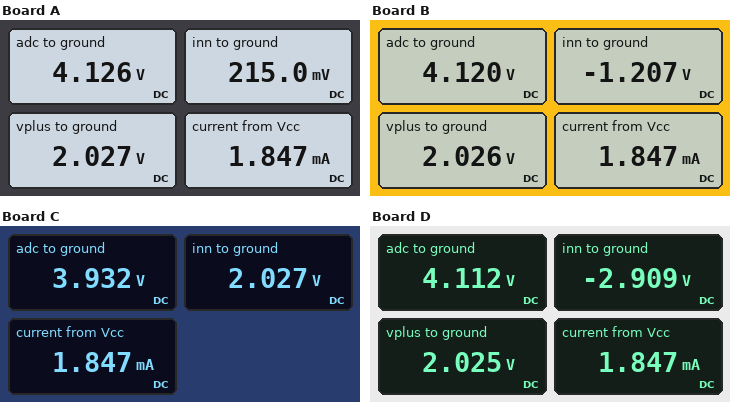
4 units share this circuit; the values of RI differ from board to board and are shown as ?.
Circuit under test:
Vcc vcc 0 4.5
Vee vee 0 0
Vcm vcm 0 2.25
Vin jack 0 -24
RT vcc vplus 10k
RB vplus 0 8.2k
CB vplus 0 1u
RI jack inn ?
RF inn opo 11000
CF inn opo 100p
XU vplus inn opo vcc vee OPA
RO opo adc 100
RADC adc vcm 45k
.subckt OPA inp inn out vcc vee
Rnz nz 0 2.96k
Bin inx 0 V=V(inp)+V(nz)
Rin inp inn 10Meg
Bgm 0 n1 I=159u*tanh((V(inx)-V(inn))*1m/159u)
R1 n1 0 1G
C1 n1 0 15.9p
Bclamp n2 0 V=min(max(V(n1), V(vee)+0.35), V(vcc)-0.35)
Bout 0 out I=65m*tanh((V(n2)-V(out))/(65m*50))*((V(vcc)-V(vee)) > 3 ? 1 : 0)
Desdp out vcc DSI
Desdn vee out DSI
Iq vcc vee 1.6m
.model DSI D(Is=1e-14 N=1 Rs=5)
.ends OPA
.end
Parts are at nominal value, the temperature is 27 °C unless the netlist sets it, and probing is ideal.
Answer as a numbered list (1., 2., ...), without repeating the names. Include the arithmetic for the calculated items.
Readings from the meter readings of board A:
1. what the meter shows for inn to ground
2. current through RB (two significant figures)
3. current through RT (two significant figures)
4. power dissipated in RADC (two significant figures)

1. 215.0 mV
2. (2.027 V) / 8.2 kΩ = 250 µA
3. (4.5 V - 2.027 V) / 10 kΩ = 250 µA
4. (4.126 V - 2.25 V)^2 / 45 kΩ = 78 µW
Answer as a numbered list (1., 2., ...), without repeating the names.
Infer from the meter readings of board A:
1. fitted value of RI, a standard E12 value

1. 68 kΩ
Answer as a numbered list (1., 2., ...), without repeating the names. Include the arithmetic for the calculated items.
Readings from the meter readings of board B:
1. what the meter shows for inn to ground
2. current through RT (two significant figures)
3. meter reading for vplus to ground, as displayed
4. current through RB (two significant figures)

1. -1.207 V
2. (4.5 V - 2.026 V) / 10 kΩ = 250 µA
3. 2.026 V
4. (2.026 V) / 8.2 kΩ = 250 µA
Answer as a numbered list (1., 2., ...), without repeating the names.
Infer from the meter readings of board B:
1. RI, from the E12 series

1. 47 kΩ
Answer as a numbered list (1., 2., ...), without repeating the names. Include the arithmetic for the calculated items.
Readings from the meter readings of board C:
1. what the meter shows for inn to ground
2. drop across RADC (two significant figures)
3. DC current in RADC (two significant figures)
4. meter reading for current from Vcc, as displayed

1. 2.027 V
2. 3.932 V - 2.25 V = 1.7 V
3. (3.932 V - 2.25 V) / 45 kΩ = 37 µA
4. 1.847 mA
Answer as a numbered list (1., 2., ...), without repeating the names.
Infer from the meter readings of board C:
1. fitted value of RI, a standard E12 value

1. 150 kΩ
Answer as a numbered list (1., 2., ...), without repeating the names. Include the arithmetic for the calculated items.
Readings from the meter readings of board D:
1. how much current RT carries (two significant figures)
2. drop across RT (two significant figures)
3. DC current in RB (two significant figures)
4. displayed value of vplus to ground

1. (4.5 V - 2.025 V) / 10 kΩ = 250 µA
2. 4.5 V - 2.025 V = 2.5 V
3. (2.025 V) / 8.2 kΩ = 250 µA
4. 2.025 V
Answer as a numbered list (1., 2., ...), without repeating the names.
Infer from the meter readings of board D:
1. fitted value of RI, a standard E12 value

1. 33 kΩ
